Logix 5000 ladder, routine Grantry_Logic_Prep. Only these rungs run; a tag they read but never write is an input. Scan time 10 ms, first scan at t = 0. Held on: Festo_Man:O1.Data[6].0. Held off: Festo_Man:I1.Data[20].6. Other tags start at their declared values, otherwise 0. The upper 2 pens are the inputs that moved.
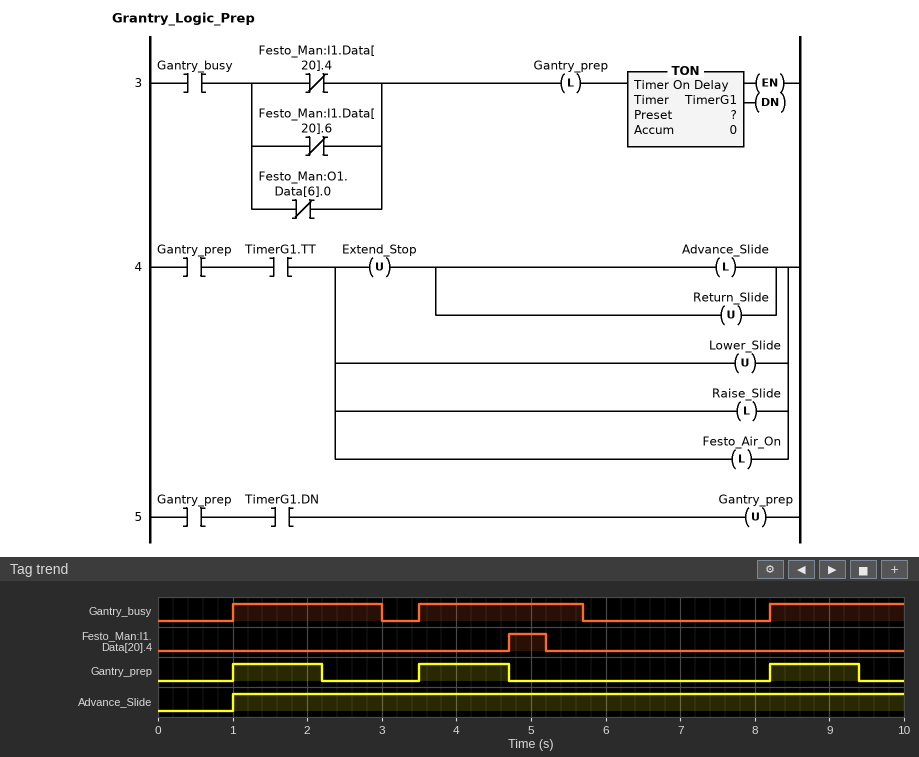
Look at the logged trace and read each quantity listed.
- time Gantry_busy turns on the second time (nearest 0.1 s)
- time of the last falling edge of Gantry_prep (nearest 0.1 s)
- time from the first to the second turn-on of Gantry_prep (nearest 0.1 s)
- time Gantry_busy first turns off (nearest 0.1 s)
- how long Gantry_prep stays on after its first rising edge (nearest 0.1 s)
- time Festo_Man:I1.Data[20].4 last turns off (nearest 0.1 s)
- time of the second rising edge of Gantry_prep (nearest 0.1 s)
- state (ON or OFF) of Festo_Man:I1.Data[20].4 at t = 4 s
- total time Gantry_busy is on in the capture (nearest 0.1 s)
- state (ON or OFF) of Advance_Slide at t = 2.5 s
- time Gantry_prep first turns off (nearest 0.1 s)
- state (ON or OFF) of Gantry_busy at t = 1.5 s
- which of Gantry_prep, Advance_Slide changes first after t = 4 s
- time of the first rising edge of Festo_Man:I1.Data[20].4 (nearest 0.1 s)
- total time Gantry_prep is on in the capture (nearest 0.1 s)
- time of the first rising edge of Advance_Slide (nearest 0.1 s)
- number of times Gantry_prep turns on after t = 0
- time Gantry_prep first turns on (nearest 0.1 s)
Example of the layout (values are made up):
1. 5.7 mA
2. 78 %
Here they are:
1. 3.5 s
2. 9.4 s
3. 2.5 s
4. 3.0 s
5. 1.2 s
6. 5.2 s
7. 3.5 s
8. OFF
9. 6.0 s
10. ON
11. 2.2 s
12. ON
13. Gantry_prep
14. 4.7 s
15. 3.6 s
16. 1.0 s
17. 3
18. 1.0 s
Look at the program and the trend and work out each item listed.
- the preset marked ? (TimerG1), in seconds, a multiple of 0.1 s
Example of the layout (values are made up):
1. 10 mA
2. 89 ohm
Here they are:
1. 1.2 s
